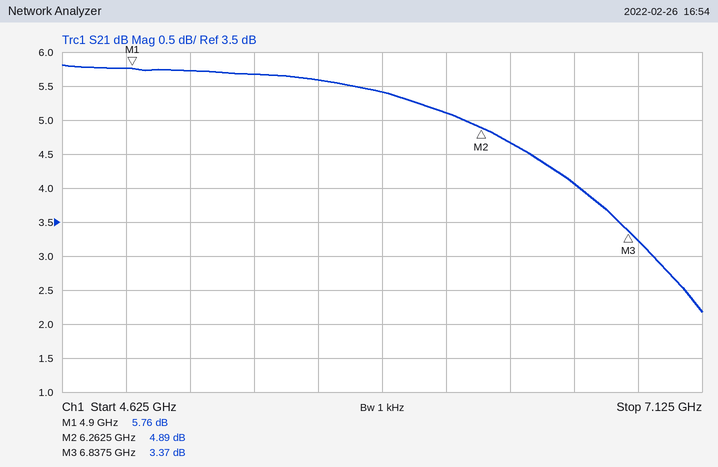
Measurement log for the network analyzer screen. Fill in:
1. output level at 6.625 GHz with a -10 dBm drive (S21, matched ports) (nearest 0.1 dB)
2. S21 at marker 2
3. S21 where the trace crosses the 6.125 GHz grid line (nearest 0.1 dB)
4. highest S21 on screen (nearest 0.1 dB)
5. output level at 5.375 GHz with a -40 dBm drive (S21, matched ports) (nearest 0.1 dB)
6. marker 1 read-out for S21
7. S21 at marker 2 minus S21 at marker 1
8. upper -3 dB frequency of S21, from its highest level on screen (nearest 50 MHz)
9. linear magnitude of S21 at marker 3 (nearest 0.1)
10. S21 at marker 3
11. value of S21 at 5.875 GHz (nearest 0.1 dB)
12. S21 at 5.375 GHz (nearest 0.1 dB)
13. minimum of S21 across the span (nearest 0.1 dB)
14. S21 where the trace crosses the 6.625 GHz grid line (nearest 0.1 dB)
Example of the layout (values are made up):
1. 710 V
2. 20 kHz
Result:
1. -5.9 dBm
2. 4.89 dB
3. 5.1 dB
4. 5.8 dB
5. -34.3 dBm
6. 5.76 dB
7. -0.87 dB
8. 7.00 GHz
9. 1.5
10. 3.37 dB
11. 5.4 dB
12. 5.7 dB
13. 2.2 dB
14. 4.1 dB
